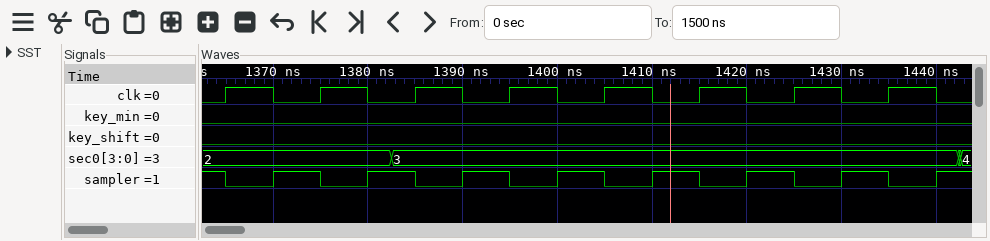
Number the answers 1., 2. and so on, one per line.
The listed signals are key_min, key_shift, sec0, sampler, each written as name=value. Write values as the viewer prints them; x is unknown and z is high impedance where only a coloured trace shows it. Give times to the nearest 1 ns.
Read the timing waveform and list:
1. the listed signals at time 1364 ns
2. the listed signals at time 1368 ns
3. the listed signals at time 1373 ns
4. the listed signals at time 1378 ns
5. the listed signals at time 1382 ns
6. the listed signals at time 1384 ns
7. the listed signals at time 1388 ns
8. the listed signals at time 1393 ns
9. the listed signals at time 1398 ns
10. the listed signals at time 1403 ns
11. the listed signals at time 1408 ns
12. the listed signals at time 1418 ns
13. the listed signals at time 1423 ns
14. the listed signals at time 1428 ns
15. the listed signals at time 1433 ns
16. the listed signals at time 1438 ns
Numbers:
1. key_min=0, key_shift=0, sec0=2, sampler=1
2. key_min=0, key_shift=0, sec0=2, sampler=0
3. key_min=0, key_shift=0, sec0=2, sampler=1
4. key_min=0, key_shift=0, sec0=2, sampler=0
5. key_min=0, key_shift=0, sec0=2, sampler=1
6. key_min=0, key_shift=0, sec0=3, sampler=1
7. key_min=0, key_shift=0, sec0=3, sampler=0
8. key_min=0, key_shift=0, sec0=3, sampler=1
9. key_min=0, key_shift=0, sec0=3, sampler=0
10. key_min=0, key_shift=0, sec0=3, sampler=1
11. key_min=0, key_shift=0, sec0=3, sampler=0
12. key_min=0, key_shift=0, sec0=3, sampler=0
13. key_min=0, key_shift=0, sec0=3, sampler=1
14. key_min=0, key_shift=0, sec0=3, sampler=0
15. key_min=0, key_shift=0, sec0=3, sampler=1
16. key_min=0, key_shift=0, sec0=3, sampler=0
